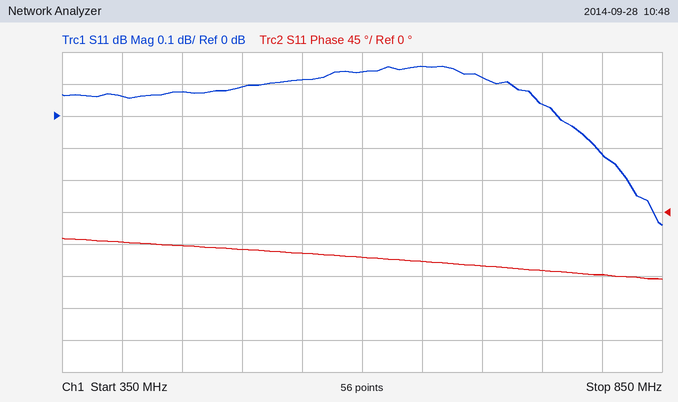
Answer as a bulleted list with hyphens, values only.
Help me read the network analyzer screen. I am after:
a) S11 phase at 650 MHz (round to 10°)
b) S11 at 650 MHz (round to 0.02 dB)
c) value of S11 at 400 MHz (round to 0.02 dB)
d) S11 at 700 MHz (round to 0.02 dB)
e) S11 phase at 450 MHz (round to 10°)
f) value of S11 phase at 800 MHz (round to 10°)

- -70°
- 0.16 dB
- 0.06 dB
- 0.12 dB
- -50°
- -90°
